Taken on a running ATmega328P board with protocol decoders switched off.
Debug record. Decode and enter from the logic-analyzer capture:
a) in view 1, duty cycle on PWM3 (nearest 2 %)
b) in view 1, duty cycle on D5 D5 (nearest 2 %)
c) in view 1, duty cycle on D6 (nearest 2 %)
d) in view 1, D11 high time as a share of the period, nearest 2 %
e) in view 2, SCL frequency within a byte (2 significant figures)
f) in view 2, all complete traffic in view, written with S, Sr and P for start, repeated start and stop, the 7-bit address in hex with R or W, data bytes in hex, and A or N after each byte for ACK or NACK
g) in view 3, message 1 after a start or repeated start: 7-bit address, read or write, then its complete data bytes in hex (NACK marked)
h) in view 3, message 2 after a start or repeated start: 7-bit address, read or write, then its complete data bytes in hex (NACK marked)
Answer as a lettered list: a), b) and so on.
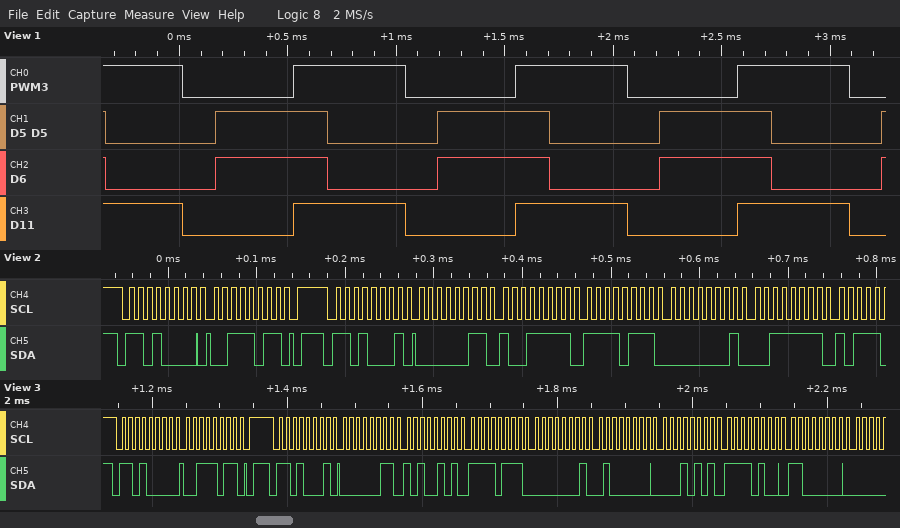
a) 50 %
b) 50 %
c) 50 %
d) 50 %
e) 100 kHz
f) S 68W A 3B A P S 68R A 03 A 9F A F7 A 01 A 3F A
g) 0x68 write: 3B
h) 0x68 read: 03 A5 F7 01 40 15 F4 C0
